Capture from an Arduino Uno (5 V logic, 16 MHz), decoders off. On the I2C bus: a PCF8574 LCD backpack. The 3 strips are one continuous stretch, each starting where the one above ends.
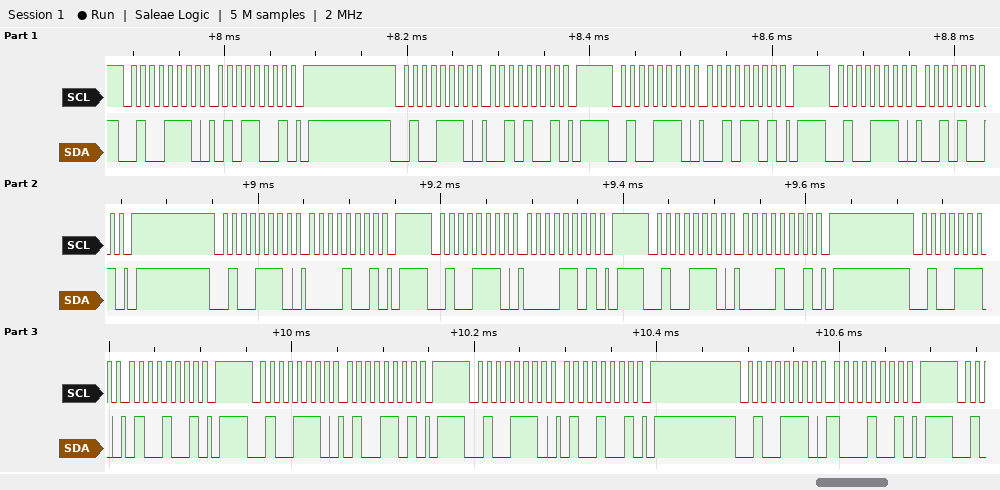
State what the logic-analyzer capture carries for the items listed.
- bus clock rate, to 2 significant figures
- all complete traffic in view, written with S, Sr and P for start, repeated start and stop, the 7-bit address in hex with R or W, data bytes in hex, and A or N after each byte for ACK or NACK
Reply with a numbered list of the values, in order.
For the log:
1. 100 kHz
2. S 27W A 59 A P S 27W A 29 A P S 27W A 2D A P S 27W A 29 A P S 27W A 09 A P S 27W A 0D A P S 27W A 09 A P S 27W A 49 A P S 27W A 4D A P S 27W A 49 A P S 27W A 89 A P
